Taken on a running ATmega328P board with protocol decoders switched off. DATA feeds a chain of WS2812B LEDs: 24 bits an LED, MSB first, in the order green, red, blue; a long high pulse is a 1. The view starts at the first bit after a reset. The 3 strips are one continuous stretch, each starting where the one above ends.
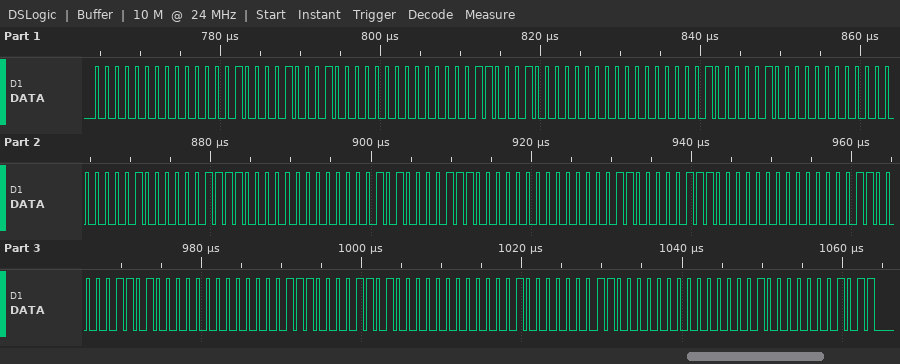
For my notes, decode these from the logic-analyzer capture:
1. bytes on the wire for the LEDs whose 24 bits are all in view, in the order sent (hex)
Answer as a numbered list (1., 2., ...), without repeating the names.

1. 00 02 11 00 03 10 00 04 10 00 04 0F 00 05 0E 00 06 0E 00 06 0D 00 07 0D 00 08 0C 00 08 0B
